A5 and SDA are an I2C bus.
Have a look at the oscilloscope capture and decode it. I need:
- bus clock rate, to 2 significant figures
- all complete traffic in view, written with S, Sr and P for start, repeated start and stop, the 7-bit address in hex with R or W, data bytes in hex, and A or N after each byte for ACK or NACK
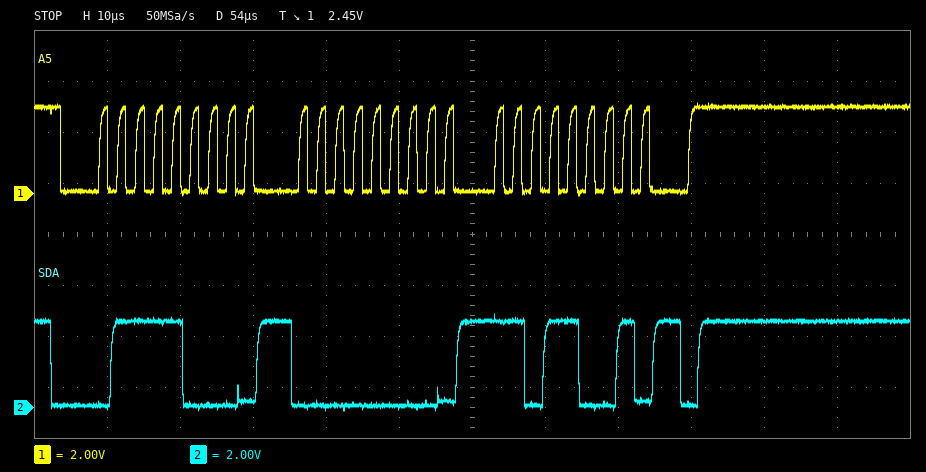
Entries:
400 kHz
S 3CW A 00 A D9 A P
